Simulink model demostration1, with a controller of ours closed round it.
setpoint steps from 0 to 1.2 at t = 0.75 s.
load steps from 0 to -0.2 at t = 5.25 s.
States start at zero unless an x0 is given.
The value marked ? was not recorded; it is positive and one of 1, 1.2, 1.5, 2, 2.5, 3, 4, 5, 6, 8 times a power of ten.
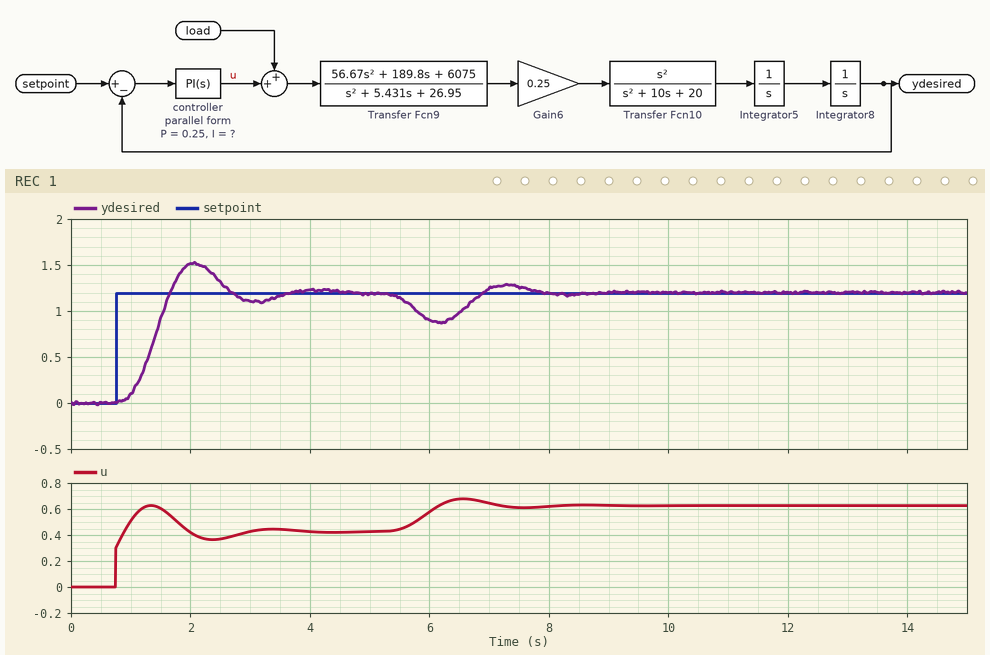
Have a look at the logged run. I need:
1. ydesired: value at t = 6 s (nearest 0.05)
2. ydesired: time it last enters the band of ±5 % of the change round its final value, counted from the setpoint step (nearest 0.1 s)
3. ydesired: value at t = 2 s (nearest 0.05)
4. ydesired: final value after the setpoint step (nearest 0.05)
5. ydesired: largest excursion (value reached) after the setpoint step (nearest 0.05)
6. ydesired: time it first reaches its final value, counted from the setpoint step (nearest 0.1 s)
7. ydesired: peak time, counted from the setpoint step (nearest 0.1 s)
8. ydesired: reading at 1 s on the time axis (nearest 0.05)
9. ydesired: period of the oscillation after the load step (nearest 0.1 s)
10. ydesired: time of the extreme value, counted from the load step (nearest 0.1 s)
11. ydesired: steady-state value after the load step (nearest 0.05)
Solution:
0.90
2.6 s
1.50
1.20
1.50
0.9 s
1.3 s
0.10
2.1 s
0.9 s
1.20
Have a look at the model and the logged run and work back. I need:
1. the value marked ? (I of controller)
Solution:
0.8
